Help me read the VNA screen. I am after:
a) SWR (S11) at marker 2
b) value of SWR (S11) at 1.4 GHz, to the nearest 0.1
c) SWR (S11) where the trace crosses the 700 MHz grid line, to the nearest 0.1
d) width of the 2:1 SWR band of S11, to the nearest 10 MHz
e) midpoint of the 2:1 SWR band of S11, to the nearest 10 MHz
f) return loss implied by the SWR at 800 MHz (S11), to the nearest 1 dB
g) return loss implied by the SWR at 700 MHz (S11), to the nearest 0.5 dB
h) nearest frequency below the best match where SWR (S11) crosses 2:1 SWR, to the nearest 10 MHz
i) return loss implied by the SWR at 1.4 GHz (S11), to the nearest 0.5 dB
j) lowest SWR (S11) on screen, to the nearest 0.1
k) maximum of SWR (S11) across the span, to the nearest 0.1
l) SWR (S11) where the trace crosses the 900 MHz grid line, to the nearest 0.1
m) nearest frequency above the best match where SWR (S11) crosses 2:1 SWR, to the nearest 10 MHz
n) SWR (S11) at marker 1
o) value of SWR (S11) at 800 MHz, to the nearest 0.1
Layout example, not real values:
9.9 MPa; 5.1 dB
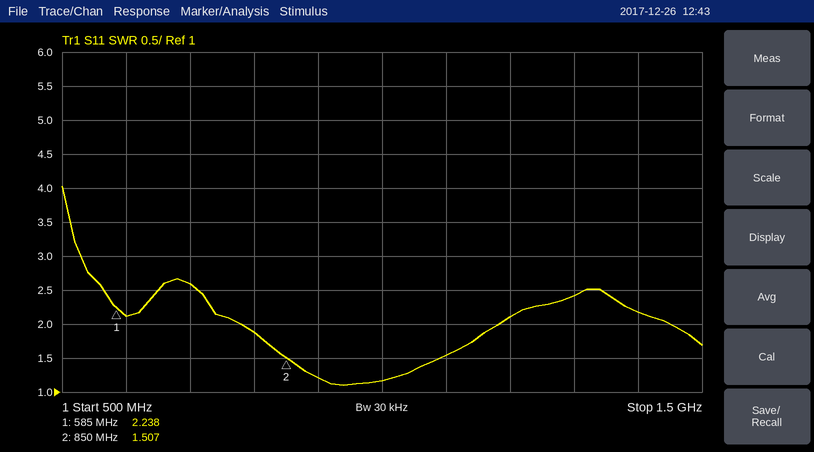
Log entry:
1.507; 2.2; 2.6; 400 MHz; 980 MHz; 10 dB; 7.0 dB; 780 MHz; 8.5 dB; 1.1; 4.0; 1.2; 1.18 GHz; 2.238; 1.9
